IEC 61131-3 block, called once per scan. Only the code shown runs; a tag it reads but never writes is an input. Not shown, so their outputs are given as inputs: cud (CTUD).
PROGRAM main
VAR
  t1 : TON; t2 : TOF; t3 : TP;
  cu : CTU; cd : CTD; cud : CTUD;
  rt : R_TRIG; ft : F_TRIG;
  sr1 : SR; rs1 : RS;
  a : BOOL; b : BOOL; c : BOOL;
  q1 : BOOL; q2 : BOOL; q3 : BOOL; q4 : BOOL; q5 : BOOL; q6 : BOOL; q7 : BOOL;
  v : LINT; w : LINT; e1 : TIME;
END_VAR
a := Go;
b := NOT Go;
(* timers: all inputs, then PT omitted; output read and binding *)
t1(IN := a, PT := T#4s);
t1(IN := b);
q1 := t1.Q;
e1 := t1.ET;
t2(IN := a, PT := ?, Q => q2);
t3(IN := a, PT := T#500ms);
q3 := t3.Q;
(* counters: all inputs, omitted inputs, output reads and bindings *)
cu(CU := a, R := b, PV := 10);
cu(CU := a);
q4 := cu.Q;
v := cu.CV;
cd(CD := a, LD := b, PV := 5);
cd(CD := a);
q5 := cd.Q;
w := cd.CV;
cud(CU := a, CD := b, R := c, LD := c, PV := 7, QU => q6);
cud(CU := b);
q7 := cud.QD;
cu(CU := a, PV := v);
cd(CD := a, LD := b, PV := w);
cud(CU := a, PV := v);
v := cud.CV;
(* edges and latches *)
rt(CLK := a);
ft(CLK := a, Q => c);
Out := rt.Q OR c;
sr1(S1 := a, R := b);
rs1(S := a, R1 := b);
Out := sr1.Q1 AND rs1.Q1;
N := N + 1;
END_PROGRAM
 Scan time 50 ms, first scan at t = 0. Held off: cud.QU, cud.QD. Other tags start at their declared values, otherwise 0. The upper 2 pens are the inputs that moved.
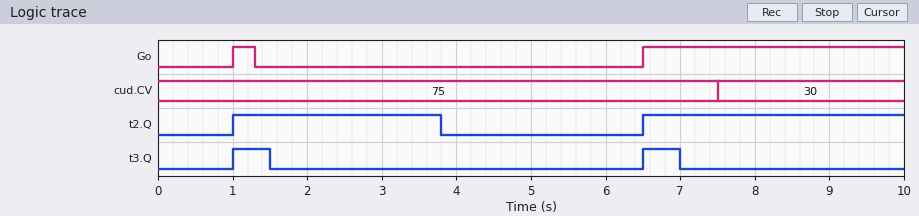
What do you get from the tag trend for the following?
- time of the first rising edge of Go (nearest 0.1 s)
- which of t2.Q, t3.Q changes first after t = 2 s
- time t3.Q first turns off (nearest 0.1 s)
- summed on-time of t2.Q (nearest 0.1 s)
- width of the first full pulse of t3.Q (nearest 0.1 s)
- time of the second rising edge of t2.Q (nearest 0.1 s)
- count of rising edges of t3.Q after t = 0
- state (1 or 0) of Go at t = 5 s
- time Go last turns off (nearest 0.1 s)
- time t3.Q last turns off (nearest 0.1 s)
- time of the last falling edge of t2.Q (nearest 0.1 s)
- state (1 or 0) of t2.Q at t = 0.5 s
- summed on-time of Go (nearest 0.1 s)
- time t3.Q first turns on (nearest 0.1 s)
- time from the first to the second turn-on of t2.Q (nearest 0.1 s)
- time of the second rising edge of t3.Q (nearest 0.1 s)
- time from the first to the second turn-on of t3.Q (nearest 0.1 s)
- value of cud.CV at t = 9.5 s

1.0 s
t2.Q
1.5 s
6.3 s
0.5 s
6.5 s
2
0
1.3 s
7.0 s
3.8 s
0
3.8 s
1.0 s
5.5 s
6.5 s
5.5 s
30
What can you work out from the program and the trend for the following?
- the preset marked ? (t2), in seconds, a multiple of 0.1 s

2.5 s
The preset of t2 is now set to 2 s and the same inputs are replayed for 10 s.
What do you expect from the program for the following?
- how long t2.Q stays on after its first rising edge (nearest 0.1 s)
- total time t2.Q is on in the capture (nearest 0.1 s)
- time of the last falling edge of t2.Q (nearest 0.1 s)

2.3 s
5.8 s
3.3 s
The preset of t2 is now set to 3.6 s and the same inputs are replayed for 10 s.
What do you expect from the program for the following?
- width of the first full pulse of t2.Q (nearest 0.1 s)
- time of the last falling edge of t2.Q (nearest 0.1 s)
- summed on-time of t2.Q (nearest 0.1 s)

3.9 s
4.9 s
7.4 s
